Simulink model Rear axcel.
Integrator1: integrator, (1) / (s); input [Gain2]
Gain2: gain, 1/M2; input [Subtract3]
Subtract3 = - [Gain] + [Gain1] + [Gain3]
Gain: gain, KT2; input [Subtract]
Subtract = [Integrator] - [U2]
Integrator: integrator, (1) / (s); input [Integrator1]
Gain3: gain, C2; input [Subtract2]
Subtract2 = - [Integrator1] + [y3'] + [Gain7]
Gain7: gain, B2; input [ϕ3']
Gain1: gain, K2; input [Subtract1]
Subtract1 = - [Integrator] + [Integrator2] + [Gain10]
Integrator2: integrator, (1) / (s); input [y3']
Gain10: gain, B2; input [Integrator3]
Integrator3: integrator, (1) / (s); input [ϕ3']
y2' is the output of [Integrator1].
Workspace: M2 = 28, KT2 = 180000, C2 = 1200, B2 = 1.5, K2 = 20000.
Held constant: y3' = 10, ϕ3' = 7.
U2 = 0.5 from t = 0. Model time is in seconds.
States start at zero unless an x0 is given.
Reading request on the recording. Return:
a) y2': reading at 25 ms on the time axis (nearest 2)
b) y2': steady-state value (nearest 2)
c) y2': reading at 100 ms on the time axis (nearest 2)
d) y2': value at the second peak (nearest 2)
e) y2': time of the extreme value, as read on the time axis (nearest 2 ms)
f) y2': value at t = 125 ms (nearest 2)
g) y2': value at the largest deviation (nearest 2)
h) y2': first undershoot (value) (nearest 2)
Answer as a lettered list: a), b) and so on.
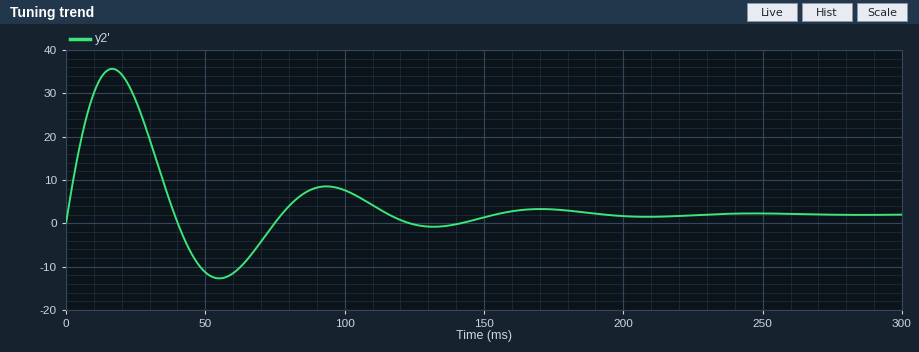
a) 28
b) 2
c) 8
d) 8
e) 16 ms
f) 0
g) 36
h) -12
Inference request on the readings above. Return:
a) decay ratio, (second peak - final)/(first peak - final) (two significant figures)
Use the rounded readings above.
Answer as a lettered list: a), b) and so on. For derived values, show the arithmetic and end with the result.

a) (8 - 2) / (36 - 2) = 0.18
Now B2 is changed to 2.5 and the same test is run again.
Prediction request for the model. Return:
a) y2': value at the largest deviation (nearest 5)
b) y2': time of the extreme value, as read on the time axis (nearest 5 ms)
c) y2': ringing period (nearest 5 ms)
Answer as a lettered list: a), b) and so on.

a) 40
b) 15 ms
c) 75 ms
